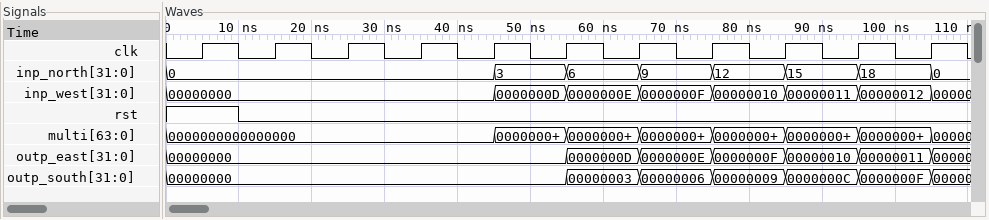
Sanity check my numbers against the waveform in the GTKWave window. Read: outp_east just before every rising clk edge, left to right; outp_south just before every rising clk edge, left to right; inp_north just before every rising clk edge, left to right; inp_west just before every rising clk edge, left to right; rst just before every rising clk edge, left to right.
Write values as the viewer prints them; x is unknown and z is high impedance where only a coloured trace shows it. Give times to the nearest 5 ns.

00000000, 00000000, 00000000, 00000000, 00000000, 00000000, 0000000D, 0000000E, 0000000F, 00000010, 00000011
00000000, 00000000, 00000000, 00000000, 00000000, 00000000, 00000003, 00000006, 00000009, 0000000C, 0000000F
0, 0, 0, 0, 0, 3, 6, 9, 12, 15, 18
00000000, 00000000, 00000000, 00000000, 00000000, 0000000D, 0000000E, 0000000F, 00000010, 00000011, 00000012
1 0 0 0 0 0 0 0 0 0 0
